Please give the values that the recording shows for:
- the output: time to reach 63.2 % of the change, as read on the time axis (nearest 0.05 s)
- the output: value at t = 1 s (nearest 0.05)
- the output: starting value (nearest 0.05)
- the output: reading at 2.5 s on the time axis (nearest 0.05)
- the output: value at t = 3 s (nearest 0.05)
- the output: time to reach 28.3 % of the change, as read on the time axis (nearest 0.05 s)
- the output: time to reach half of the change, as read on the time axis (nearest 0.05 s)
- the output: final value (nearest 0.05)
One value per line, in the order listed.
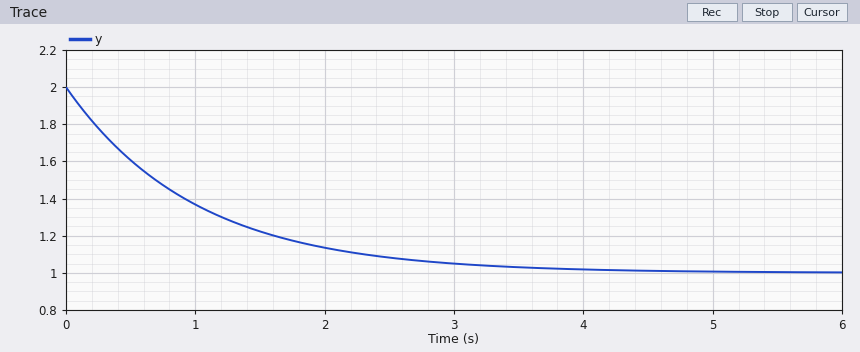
1.00 s
1.35
2.00
1.10
1.05
0.35 s
0.70 s
1.00
